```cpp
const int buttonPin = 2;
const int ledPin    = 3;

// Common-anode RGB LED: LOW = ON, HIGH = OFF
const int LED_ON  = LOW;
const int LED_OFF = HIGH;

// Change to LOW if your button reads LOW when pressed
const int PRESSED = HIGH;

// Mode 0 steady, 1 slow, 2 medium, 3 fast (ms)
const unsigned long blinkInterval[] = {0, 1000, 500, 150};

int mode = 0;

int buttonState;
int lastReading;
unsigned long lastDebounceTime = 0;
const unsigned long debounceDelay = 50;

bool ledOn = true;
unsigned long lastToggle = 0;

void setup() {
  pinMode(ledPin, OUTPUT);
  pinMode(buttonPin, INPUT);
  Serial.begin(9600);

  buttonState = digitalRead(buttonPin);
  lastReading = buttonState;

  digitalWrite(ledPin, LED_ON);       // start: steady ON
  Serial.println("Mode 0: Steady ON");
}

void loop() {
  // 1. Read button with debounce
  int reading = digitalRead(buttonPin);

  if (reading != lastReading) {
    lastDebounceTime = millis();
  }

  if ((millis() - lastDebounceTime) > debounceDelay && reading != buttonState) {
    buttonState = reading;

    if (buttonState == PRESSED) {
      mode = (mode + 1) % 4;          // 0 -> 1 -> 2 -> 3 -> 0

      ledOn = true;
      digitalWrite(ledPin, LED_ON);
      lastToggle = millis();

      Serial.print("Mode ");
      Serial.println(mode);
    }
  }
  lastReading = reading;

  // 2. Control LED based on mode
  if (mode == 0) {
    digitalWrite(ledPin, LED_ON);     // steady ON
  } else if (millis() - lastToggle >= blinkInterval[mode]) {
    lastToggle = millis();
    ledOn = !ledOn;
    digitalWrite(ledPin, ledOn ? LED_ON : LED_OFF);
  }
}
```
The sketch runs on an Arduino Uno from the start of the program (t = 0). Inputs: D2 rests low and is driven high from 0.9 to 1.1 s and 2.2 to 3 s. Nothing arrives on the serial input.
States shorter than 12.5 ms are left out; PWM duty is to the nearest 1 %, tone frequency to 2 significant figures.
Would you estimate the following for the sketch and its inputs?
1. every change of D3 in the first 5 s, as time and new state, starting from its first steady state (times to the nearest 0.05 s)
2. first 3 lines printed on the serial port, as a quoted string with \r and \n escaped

0 s low; 1.95 s high; 2.25 s low; 2.75 s high; 3.25 s low; 3.75 s high; 4.25 s low; 4.75 s high
"Mode 0: Steady ON\r\nMode 1\r\nMode 2\r\n"
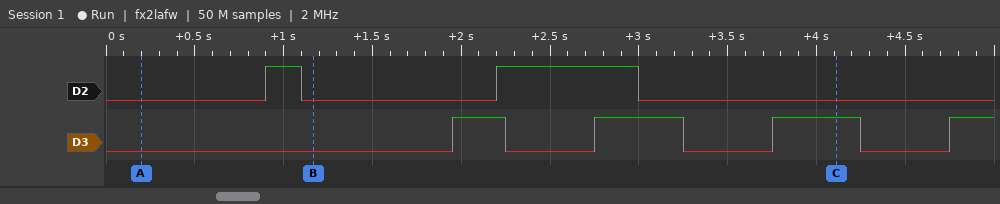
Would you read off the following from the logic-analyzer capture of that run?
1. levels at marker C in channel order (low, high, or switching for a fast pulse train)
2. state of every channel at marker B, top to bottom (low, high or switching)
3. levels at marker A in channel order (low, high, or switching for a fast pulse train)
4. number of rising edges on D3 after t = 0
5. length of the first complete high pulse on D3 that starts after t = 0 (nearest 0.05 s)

D2 low, D3 high
D2 low, D3 low
D2 low, D3 low
4
0.30 s
